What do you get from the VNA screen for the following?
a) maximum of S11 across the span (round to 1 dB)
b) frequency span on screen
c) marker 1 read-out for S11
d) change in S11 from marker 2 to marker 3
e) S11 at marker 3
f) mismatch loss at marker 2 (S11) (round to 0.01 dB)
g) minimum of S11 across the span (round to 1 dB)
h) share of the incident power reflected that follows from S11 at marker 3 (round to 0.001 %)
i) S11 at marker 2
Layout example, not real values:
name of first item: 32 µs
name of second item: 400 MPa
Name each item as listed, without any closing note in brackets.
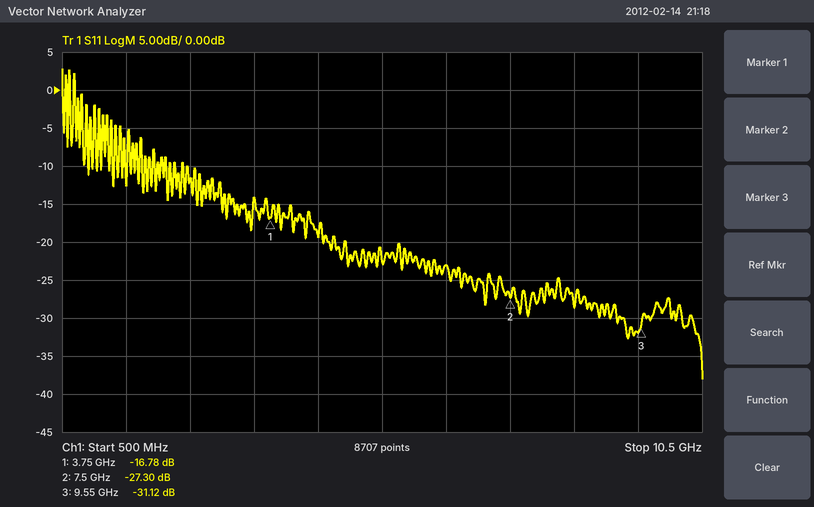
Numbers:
maximum of S11 across the span: 3 dB
frequency span on screen: 10 GHz
marker 1 read-out for S11: -16.78 dB
change in S11 from marker 2 to marker 3: -3.82 dB
S11 at marker 3: -31.12 dB
mismatch loss at marker 2 (S11): 0.01 dB
minimum of S11 across the span: -38 dB
share of the incident power reflected that follows from S11 at marker 3: 0.077 %
S11 at marker 2: -27.30 dB
